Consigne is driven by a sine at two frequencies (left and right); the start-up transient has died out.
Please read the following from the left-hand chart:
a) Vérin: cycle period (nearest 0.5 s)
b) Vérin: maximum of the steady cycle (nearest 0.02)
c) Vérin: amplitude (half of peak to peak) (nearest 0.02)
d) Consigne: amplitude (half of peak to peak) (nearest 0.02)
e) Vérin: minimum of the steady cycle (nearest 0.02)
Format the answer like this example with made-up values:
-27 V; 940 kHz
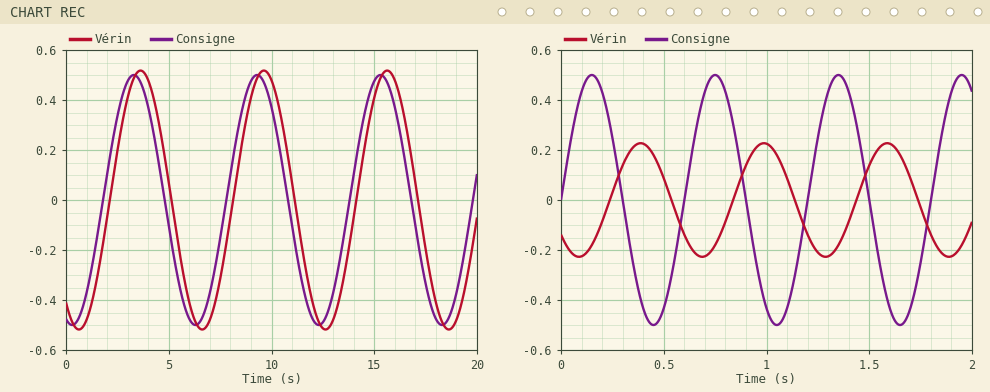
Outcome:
6.0 s; 0.52; 0.52; 0.50; -0.52
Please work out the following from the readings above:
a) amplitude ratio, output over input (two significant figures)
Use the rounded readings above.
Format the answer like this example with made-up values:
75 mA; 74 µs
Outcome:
1.0
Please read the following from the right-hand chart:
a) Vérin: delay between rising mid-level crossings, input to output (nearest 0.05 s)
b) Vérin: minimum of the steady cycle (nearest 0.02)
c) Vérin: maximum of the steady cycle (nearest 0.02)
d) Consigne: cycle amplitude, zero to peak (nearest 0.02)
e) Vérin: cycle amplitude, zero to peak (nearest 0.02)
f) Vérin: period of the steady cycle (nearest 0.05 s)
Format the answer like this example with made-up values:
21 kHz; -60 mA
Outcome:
0.25 s; -0.22; 0.22; 0.50; 0.22; 0.60 s
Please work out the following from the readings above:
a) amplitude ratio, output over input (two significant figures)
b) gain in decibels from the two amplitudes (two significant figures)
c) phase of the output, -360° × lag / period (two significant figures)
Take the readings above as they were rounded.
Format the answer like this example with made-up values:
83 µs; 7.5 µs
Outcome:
0.44; -7.1 dB; -150°
